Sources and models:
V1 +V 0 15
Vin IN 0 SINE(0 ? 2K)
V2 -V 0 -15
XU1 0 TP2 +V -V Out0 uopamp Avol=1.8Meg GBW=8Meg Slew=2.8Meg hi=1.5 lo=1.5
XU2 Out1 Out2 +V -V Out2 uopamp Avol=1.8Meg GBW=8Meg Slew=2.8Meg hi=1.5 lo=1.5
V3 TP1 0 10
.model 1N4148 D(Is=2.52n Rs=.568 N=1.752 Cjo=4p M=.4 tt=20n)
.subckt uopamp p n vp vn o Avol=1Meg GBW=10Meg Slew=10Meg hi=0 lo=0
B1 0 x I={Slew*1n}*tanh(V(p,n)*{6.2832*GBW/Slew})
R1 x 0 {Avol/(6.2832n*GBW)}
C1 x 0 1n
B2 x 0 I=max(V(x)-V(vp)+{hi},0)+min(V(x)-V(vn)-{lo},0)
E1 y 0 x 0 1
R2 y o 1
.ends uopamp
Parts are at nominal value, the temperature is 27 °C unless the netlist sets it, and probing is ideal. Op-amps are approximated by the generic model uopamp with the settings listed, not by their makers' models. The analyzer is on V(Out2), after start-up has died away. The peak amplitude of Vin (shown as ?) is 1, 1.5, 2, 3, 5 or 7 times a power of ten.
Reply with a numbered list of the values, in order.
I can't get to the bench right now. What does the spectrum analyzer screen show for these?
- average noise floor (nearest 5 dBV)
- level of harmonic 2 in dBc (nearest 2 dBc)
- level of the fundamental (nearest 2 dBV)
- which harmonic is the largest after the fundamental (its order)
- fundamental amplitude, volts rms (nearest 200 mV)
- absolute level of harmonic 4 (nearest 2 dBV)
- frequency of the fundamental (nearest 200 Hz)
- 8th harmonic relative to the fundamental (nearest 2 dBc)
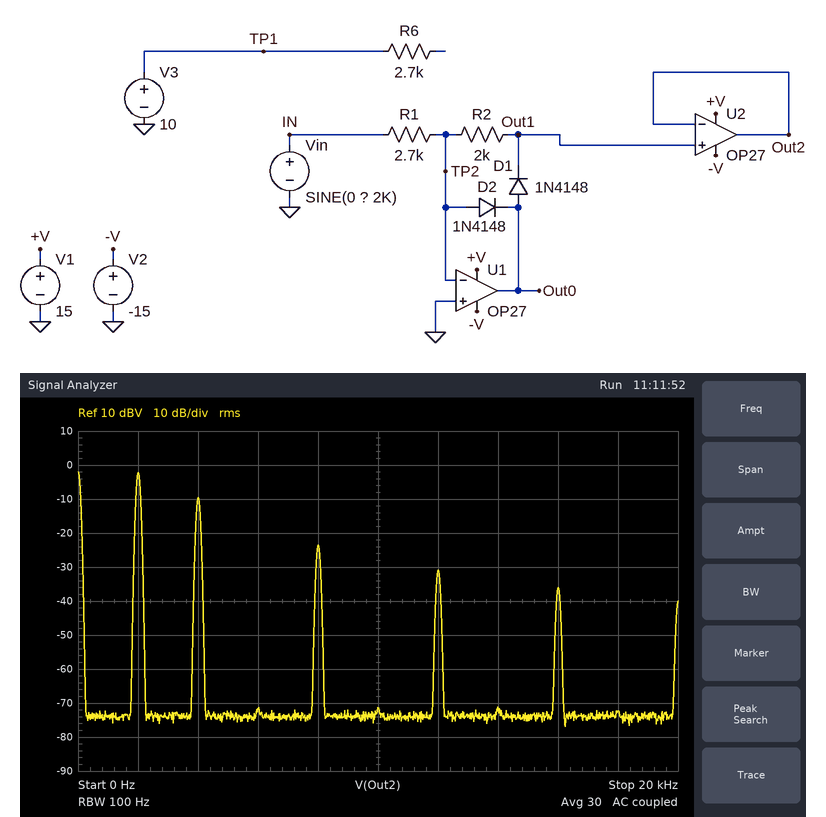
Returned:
1. -75 dBV
2. -8 dBc
3. -2 dBV
4. 2
5. 800 mV
6. -24 dBV
7. 2.0 kHz
8. -34 dBc
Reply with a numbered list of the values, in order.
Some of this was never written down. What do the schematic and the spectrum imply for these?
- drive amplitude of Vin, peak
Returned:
1. 3 V
